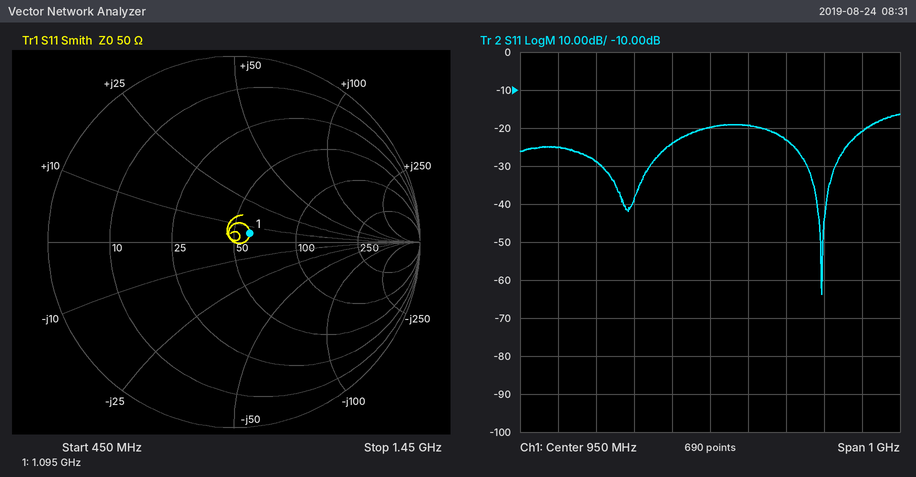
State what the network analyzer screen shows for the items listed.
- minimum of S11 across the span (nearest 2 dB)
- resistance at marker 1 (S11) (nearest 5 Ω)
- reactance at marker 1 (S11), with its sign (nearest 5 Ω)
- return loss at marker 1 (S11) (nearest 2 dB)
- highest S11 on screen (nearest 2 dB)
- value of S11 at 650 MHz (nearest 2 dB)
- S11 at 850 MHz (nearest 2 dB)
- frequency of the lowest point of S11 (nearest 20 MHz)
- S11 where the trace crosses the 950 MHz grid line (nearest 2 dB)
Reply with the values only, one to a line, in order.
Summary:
-64 dB
60 Ω
+5 Ω
20 dB
-16 dB
-28 dB
-24 dB
1.24 GHz
-20 dB
